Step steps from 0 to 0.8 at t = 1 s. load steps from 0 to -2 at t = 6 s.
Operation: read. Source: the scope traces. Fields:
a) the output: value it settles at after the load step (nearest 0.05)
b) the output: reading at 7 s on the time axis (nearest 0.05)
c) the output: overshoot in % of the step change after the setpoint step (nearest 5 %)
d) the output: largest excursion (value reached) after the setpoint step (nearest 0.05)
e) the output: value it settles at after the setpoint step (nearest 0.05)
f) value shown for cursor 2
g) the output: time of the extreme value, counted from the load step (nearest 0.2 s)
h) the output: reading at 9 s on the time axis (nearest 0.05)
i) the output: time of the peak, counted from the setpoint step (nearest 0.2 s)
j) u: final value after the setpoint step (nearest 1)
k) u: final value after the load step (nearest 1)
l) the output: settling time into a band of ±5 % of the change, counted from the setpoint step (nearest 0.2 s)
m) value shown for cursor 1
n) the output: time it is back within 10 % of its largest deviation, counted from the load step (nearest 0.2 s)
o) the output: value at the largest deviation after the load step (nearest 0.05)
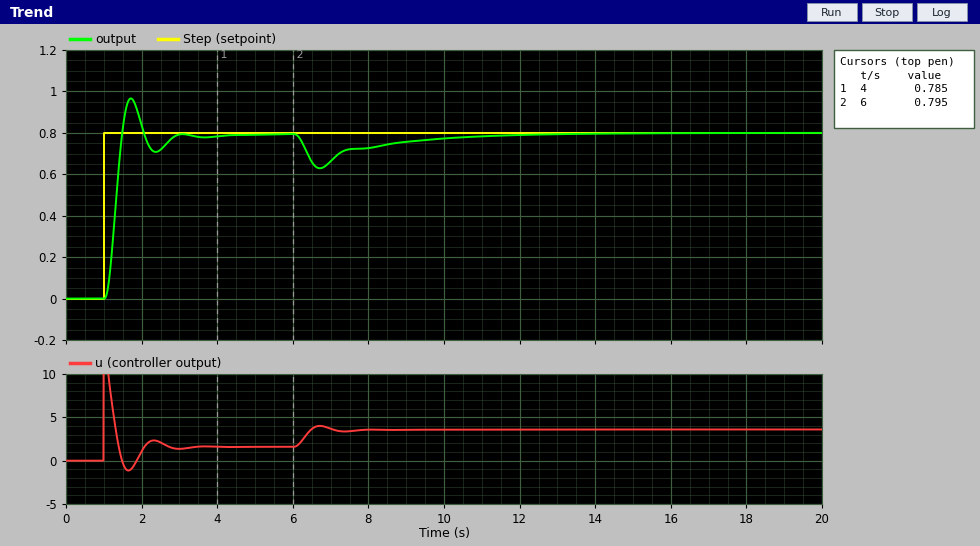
0.80
0.65
20 %
0.95
0.80
0.795
0.8 s
0.75
0.8 s
2
4
1.8 s
0.785
5.0 s
0.65
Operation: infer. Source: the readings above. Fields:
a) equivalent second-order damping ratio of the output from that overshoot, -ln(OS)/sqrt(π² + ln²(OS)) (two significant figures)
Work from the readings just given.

0.46
